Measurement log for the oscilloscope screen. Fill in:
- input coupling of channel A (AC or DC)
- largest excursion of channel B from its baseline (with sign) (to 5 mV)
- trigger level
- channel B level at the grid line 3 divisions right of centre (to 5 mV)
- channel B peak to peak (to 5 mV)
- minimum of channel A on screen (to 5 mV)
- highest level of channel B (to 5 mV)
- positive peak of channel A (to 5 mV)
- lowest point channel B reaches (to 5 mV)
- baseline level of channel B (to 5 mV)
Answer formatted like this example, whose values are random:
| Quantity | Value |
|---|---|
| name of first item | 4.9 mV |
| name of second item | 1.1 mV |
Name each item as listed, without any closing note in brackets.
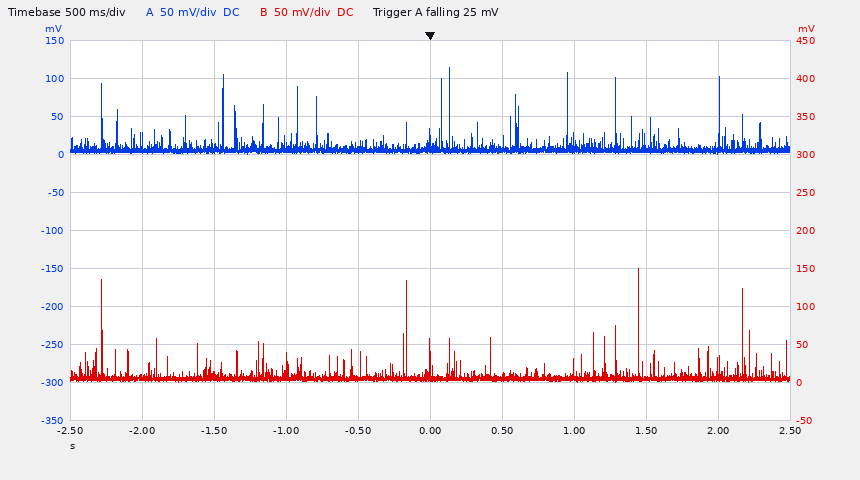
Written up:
| Quantity | Value |
|---|---|
| input coupling of channel A | DC |
| largest excursion of channel B from its baseline (with sign) | +145 mV |
| trigger level | 25 mV |
| channel B level at the grid line 3 divisions right of centre | 5 mV |
| channel B peak to peak | 150 mV |
| minimum of channel A on screen | 0 mV |
| highest level of channel B | 150 mV |
| positive peak of channel A | 115 mV |
| lowest point channel B reaches | 0 mV |
| baseline level of channel B | 5 mV |
